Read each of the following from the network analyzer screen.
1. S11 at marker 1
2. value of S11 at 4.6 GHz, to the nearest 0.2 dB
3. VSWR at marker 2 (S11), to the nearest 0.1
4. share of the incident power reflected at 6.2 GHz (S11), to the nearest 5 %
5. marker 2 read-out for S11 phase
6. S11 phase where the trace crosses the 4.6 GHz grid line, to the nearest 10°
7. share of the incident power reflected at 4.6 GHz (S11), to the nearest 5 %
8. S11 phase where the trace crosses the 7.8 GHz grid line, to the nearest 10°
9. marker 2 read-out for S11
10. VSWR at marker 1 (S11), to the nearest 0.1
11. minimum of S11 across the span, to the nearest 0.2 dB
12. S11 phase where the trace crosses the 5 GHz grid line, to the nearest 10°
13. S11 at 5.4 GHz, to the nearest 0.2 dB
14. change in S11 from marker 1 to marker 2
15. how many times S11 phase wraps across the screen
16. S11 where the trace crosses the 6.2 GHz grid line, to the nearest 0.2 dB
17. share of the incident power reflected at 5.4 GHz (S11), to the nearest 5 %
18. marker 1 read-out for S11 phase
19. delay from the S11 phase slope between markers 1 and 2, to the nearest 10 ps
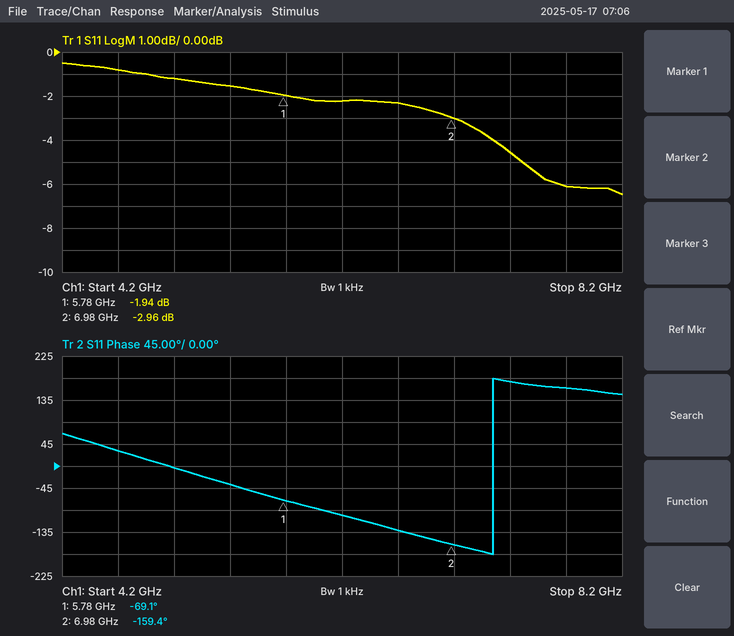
-1.94 dB
-0.8 dB
5.9
60 %
-159.4°
30°
85 %
160°
-2.96 dB
9.0
-6.4 dB
0°
-1.6 dB
-1.02 dB
1
-2.2 dB
70 %
-69.1°
210 ps
